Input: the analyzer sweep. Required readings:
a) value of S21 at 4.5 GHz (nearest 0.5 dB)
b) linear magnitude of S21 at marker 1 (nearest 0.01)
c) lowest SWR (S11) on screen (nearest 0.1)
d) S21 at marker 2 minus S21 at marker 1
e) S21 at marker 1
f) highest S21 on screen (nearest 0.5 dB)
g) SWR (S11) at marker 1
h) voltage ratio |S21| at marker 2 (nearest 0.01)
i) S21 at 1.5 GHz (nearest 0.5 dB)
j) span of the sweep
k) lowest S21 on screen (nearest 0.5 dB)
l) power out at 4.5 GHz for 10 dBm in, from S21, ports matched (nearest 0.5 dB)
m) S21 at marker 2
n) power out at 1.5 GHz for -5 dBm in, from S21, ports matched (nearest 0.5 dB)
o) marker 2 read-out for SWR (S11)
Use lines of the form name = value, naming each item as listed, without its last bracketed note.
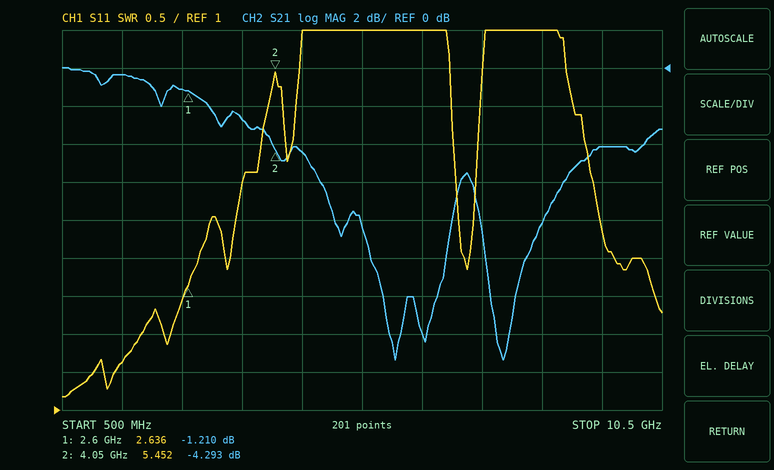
value of S21 at 4.5 GHz = -4.5 dB
linear magnitude of S21 at marker 1 = 0.87
lowest SWR (S11) on screen = 1.2
S21 at marker 2 minus S21 at marker 1 = -3.083 dB
S21 at marker 1 = -1.210 dB
highest S21 on screen = 0.0 dB
SWR (S11) at marker 1 = 2.636
voltage ratio |S21| at marker 2 = 0.61
S21 at 1.5 GHz = -0.5 dB
span of the sweep = 10 GHz
lowest S21 on screen = -15.5 dB
power out at 4.5 GHz for 10 dBm in, from S21, ports matched = 5.5 dBm
S21 at marker 2 = -4.293 dB
power out at 1.5 GHz for -5 dBm in, from S21, ports matched = -5.5 dBm
marker 2 read-out for SWR = 5.452
